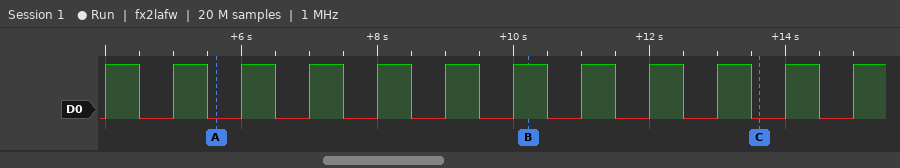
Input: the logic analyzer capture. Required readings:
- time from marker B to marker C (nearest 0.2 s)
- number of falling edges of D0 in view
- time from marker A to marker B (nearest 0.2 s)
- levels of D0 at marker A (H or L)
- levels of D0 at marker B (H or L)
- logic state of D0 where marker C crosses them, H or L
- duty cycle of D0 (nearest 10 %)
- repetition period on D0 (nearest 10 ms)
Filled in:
3.4 s
11
4.6 s
D0=L
D0=H
D0=L
50 %
1000 ms
